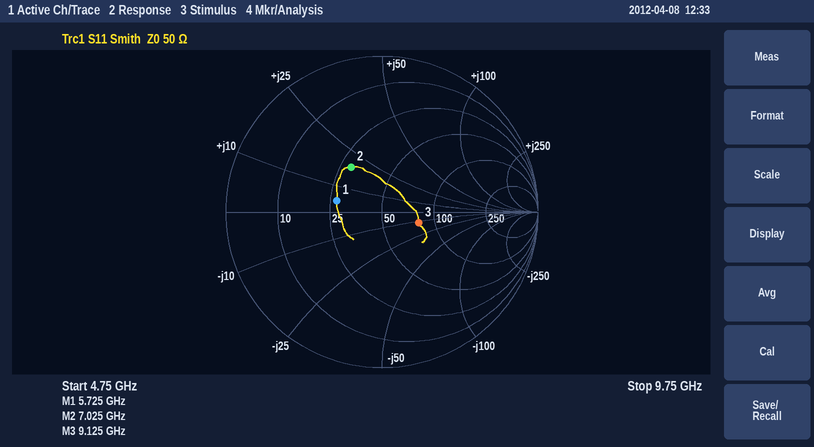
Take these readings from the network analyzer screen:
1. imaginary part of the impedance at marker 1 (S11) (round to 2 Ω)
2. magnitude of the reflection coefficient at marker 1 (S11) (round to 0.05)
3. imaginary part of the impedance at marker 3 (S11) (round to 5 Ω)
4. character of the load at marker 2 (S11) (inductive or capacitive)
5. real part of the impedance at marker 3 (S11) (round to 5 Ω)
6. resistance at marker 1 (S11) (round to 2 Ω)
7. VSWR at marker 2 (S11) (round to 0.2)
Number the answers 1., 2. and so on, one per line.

1. +4 Ω
2. 0.30
3. -10 Ω
4. inductive
5. 80 Ω
6. 28 Ω
7. 2.0
